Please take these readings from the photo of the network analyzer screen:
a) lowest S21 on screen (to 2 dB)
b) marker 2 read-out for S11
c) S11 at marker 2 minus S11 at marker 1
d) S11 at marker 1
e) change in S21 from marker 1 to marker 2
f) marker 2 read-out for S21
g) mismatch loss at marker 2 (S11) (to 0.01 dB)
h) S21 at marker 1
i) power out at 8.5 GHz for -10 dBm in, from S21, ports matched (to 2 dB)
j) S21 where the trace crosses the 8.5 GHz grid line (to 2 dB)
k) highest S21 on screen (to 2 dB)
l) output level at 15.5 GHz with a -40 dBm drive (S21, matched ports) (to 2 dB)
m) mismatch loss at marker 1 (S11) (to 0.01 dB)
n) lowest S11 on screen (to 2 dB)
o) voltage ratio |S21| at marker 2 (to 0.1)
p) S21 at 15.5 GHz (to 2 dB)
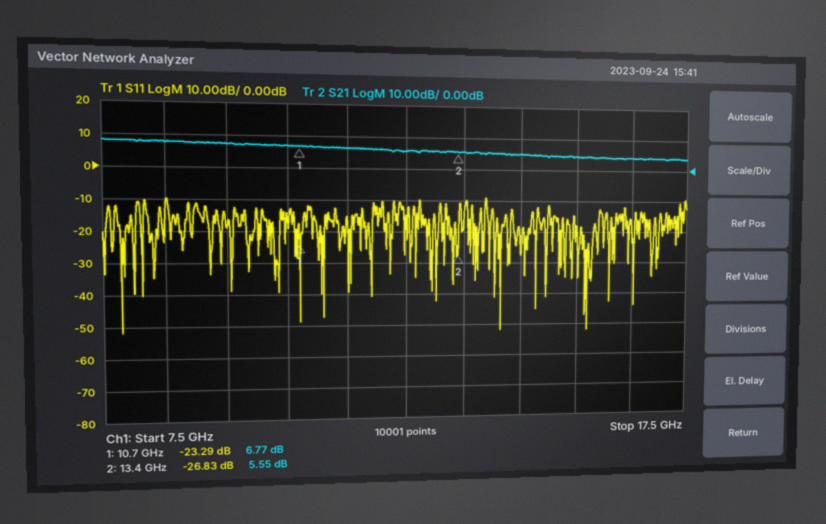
4 dB
-26.83 dB
-3.54 dB
-23.29 dB
-1.22 dB
5.55 dB
0.01 dB
6.77 dB
-2 dBm
8 dB
8 dB
-36 dBm
0.02 dB
-52 dB
1.9
4 dB
